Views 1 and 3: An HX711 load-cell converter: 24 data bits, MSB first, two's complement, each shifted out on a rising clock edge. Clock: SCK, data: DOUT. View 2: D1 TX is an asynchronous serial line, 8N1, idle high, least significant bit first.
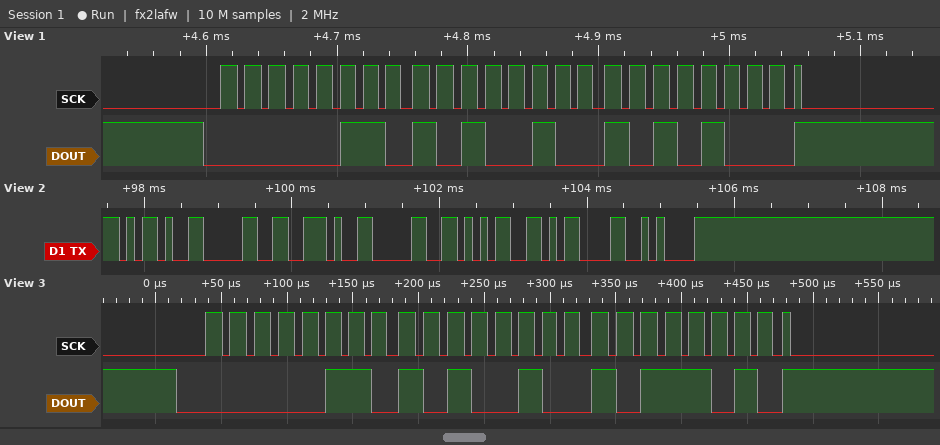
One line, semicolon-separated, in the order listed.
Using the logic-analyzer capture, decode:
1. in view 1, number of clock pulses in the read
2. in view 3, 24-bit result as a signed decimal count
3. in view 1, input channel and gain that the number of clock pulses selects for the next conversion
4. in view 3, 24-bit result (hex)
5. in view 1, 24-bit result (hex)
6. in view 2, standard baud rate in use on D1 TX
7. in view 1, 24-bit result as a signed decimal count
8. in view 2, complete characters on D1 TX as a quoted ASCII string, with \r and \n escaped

25; 435386; channel A, gain 128; 0x06A4BA; 0x06A4A8; 9600 baud; 435368; "-0.05\r\n"
